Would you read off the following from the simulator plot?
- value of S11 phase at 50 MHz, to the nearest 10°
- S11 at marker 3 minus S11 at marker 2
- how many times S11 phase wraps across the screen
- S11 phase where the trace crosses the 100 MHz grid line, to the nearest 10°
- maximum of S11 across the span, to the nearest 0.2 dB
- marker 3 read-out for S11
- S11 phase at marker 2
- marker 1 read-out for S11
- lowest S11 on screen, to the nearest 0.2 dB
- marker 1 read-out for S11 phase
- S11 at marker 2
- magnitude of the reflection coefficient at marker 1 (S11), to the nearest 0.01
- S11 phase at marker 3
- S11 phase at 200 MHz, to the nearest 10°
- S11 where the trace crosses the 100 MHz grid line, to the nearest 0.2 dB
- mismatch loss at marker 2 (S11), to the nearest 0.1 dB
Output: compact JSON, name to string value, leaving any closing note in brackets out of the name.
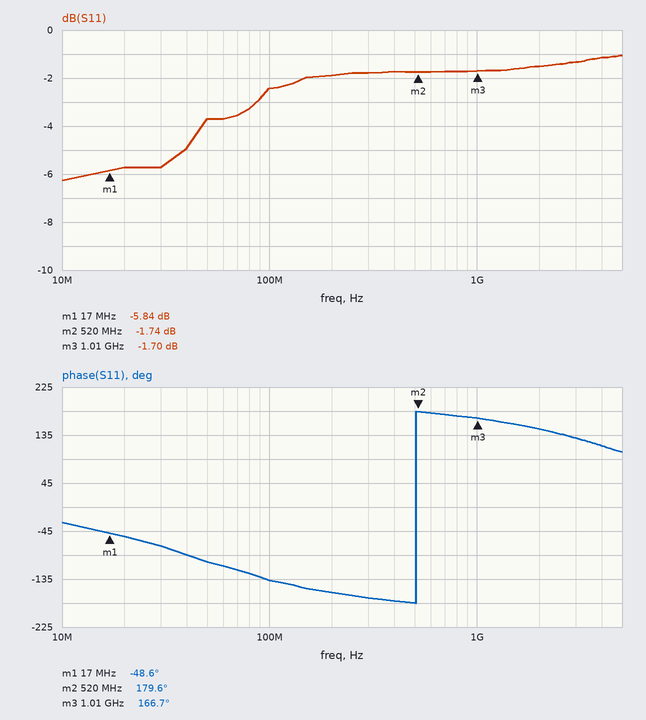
{"value of S11 phase at 50 MHz, to the nearest 10°": "-100°", "S11 at marker 3 minus S11 at marker 2": "0.04 dB", "how many times S11 phase wraps across the screen": "1", "S11 phase where the trace crosses the 100 MHz grid line, to the nearest 10°": "-140°", "maximum of S11 across the span, to the nearest 0.2 dB": "-1.0 dB", "marker 3 read-out for S11": "-1.70 dB", "S11 phase at marker 2": "179.6°", "marker 1 read-out for S11": "-5.84 dB", "lowest S11 on screen, to the nearest 0.2 dB": "-6.2 dB", "marker 1 read-out for S11 phase": "-48.6°", "S11 at marker 2": "-1.74 dB", "magnitude of the reflection coefficient at marker 1 (S11), to the nearest 0.01": "0.51", "S11 phase at marker 3": "166.7°", "S11 phase at 200 MHz, to the nearest 10°": "-160°", "S11 where the trace crosses the 100 MHz grid line, to the nearest 0.2 dB": "-2.4 dB", "mismatch loss at marker 2 (S11), to the nearest 0.1 dB": "4.8 dB"}
